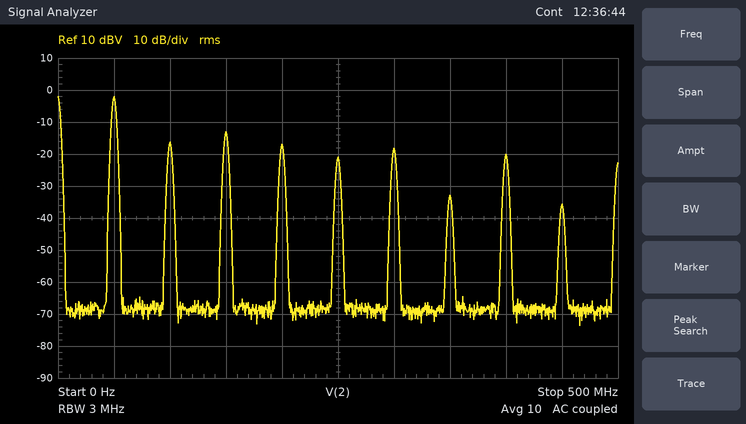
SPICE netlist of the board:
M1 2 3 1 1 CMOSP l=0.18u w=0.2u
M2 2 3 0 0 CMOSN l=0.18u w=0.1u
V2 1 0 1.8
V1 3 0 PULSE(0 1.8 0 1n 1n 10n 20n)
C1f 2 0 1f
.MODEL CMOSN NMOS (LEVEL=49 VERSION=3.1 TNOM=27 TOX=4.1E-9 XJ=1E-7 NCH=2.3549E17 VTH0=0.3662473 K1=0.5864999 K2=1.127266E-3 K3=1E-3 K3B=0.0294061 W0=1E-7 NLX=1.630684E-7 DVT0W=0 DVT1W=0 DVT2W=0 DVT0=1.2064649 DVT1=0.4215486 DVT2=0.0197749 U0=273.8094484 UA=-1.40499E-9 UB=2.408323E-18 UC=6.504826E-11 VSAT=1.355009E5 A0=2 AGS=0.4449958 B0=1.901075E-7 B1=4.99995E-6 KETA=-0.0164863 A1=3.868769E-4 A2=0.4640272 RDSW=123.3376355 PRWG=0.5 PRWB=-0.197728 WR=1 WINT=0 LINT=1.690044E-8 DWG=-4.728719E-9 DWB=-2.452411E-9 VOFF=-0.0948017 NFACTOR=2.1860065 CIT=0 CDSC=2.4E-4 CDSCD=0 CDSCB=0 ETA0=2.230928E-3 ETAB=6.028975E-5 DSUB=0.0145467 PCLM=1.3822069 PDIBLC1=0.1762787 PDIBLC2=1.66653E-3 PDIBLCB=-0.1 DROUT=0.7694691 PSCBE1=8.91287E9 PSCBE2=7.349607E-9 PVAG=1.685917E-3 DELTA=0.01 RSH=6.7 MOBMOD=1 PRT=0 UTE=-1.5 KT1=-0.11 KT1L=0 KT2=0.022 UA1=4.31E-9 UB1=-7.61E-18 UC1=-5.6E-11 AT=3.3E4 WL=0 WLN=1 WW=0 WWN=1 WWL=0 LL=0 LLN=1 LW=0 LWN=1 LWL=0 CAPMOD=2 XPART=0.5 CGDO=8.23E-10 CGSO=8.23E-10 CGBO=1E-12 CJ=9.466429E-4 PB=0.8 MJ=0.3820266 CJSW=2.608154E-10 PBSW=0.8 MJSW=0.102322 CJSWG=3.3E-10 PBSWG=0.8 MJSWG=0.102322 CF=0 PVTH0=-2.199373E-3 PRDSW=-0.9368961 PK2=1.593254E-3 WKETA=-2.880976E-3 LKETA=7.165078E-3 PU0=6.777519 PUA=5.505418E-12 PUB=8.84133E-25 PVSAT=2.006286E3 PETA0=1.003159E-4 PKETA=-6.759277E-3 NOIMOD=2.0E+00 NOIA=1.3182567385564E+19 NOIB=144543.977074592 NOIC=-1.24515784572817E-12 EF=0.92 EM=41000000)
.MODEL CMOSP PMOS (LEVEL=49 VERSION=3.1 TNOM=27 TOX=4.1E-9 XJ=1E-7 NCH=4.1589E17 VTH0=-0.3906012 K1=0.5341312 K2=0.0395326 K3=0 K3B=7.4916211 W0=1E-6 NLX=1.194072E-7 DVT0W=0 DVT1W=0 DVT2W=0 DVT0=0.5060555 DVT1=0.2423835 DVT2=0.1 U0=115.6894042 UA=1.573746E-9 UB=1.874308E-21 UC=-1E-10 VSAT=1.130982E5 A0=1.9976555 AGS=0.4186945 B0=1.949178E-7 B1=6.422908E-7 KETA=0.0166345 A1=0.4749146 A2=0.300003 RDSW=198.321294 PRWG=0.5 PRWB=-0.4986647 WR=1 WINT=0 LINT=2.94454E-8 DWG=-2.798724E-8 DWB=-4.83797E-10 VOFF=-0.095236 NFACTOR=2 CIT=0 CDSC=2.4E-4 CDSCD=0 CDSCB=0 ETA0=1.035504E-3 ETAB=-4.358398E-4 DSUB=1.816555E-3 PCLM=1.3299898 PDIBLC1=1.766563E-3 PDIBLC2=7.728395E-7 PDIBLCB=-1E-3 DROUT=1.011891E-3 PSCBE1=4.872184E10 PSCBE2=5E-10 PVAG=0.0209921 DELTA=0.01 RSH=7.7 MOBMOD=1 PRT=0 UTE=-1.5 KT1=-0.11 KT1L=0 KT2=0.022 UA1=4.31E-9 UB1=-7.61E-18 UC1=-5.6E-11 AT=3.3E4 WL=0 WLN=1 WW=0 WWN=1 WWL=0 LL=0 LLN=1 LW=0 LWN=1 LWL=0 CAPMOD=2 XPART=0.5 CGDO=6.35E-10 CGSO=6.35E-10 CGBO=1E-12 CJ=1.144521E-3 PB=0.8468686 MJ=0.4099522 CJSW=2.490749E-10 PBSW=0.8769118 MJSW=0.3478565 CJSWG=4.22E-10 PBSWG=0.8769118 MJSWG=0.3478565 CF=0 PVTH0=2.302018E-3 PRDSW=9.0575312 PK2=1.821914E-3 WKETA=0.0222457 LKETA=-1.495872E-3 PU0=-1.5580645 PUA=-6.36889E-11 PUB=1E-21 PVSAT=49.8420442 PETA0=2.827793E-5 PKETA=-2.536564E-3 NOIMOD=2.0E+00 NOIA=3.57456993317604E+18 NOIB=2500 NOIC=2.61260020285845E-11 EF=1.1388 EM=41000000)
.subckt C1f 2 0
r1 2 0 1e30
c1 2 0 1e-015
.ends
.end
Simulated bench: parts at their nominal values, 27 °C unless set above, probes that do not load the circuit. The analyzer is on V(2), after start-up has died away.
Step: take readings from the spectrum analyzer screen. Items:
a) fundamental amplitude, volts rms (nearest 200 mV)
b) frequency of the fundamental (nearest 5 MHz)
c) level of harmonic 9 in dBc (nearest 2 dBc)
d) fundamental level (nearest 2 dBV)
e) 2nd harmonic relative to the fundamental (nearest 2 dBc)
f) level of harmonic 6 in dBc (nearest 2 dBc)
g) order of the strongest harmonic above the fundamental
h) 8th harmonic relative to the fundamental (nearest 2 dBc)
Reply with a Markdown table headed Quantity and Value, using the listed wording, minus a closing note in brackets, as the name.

| Quantity | Value |
|---|---|
| fundamental amplitude, volts rms | 800 mV |
| frequency of the fundamental | 50 MHz |
| level of harmonic 9 in dBc | -34 dBc |
| fundamental level | -2 dBV |
| 2nd harmonic relative to the fundamental | -14 dBc |
| level of harmonic 6 in dBc | -16 dBc |
| order of the strongest harmonic above the fundamental | 3 |
| 8th harmonic relative to the fundamental | -18 dBc |
